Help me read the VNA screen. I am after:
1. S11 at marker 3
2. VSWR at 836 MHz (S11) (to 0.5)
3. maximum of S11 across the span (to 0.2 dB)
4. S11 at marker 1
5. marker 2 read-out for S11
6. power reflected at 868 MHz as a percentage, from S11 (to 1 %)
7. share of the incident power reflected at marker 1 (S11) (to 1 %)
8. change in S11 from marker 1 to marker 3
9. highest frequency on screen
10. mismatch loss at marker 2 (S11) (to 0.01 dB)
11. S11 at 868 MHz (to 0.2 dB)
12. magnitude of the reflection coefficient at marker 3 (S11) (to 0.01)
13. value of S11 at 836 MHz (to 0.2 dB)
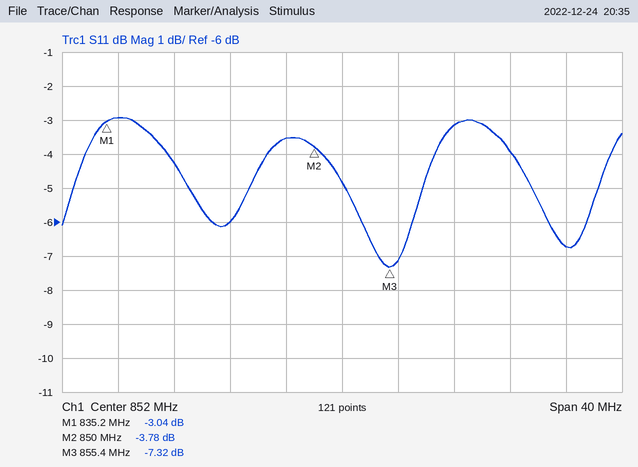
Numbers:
-7.32 dB
6.0
-3.0 dB
-3.04 dB
-3.78 dB
21 %
50 %
-4.28 dB
872 MHz
2.36 dB
-6.8 dB
0.43
-3.0 dB
